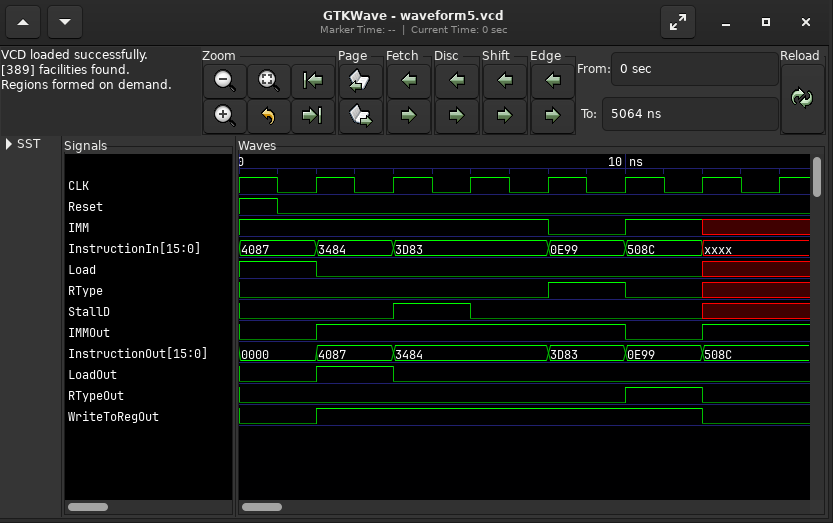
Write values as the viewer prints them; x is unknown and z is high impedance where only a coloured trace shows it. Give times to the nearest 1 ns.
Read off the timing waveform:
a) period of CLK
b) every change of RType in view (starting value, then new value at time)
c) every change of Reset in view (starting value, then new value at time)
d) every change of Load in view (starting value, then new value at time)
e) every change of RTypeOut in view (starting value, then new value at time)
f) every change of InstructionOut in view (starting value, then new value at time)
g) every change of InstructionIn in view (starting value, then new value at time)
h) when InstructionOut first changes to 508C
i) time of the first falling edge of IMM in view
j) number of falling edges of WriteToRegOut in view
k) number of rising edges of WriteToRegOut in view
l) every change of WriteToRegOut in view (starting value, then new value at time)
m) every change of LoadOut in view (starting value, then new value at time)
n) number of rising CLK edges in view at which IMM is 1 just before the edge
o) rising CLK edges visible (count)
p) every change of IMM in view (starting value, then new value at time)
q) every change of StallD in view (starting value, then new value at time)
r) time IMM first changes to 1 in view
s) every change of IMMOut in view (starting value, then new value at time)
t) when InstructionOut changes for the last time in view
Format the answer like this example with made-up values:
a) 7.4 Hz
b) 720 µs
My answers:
a) 2 ns
b) 0, 1 at 8 ns, 0 at 10 ns, x at 12 ns
c) 1, 0 at 1 ns
d) 1, 0 at 2 ns, x at 12 ns
e) 0, 1 at 10 ns, 0 at 12 ns
f) 0000, 4087 at 2 ns, 3484 at 4 ns, 3D83 at 8 ns, 0E99 at 10 ns, 508C at 12 ns
g) 4087, 3484 at 2 ns, 3D83 at 4 ns, 0E99 at 8 ns, 508C at 10 ns, xxxx at 12 ns
h) 12 ns
i) 8 ns
j) 1
k) 1
l) 0, 1 at 2 ns, 0 at 12 ns
m) 0, 1 at 2 ns, 0 at 4 ns
n) 5
o) 7
p) 1, 0 at 8 ns, 1 at 10 ns, x at 12 ns
q) 0, 1 at 4 ns, 0 at 6 ns, x at 12 ns
r) 10 ns
s) 0, 1 at 2 ns, 0 at 10 ns, 1 at 12 ns
t) 12 ns
